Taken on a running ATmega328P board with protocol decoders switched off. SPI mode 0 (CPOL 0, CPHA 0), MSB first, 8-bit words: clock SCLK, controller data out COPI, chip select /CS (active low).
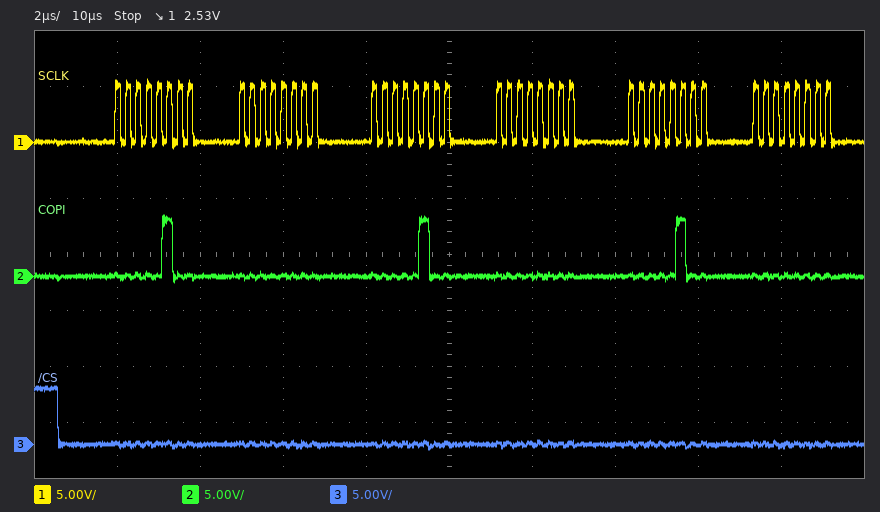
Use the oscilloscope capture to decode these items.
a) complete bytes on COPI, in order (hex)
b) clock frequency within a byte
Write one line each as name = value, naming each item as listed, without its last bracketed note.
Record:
complete bytes on COPI, in order = 0x04 0x00 0x04 0x00 0x04 0x00
clock frequency within a byte = 4 MHz
